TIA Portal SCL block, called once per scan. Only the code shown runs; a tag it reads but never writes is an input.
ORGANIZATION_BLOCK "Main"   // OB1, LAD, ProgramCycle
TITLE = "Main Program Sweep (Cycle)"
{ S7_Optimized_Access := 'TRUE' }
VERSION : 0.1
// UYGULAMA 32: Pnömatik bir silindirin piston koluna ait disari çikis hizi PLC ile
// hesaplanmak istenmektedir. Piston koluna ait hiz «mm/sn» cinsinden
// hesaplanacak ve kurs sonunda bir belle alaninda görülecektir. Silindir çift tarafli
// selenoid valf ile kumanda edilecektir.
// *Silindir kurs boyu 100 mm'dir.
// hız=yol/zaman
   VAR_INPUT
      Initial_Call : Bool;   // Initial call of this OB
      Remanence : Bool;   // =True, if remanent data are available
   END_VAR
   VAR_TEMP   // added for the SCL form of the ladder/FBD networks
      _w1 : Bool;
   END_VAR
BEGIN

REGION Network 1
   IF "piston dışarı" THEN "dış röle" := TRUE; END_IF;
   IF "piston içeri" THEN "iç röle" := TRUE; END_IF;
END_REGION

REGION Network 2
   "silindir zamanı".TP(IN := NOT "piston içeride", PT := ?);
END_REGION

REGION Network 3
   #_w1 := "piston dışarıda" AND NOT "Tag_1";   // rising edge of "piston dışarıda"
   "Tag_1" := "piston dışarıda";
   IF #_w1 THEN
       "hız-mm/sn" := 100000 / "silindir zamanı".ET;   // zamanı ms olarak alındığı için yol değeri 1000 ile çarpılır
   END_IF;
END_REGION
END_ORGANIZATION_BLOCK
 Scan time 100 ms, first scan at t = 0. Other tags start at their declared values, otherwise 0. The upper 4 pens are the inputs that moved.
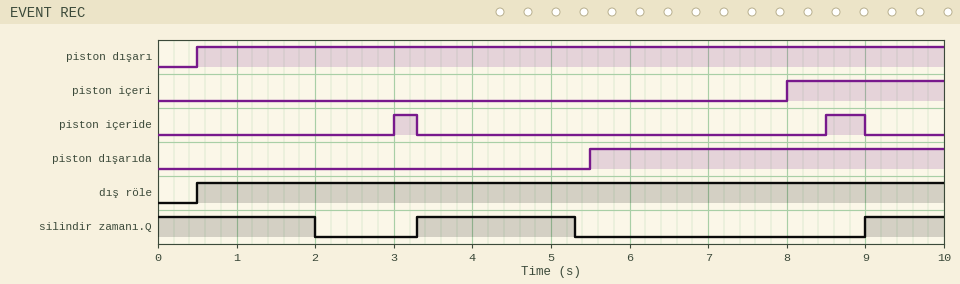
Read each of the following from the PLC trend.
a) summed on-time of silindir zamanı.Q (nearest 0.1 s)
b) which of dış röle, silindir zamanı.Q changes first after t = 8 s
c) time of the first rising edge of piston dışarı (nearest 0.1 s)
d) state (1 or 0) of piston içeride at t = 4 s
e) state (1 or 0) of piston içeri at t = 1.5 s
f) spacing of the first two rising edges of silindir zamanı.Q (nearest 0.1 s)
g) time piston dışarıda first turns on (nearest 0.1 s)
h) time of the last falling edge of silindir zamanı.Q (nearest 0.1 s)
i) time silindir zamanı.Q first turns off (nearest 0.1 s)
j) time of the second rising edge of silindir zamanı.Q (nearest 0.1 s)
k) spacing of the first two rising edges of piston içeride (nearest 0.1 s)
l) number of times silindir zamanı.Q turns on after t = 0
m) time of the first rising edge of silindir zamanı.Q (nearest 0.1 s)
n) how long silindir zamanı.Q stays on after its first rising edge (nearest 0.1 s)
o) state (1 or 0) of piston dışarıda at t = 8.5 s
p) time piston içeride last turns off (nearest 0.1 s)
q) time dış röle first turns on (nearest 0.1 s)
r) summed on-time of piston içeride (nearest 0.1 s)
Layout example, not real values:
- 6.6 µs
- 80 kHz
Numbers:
- 5.0 s
- silindir zamanı.Q
- 0.5 s
- 0
- 0
- 5.7 s
- 5.5 s
- 5.3 s
- 2.0 s
- 9.0 s
- 5.5 s
- 2
- 3.3 s
- 2.0 s
- 1
- 9.0 s
- 0.5 s
- 0.8 s
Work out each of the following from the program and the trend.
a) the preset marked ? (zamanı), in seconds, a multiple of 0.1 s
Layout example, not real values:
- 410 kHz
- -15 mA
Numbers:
- 2.0 s
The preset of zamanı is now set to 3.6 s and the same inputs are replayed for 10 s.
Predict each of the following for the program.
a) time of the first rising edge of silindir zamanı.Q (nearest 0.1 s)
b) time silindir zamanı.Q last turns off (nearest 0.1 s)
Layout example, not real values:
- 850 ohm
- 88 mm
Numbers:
- 9.0 s
- 3.6 s
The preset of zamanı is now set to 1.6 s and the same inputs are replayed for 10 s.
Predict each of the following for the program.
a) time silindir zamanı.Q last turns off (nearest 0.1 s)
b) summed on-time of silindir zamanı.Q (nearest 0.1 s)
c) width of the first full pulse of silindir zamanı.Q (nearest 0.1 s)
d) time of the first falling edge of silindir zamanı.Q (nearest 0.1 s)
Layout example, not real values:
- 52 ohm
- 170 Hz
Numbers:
- 4.9 s
- 4.2 s
- 1.6 s
- 1.6 s
